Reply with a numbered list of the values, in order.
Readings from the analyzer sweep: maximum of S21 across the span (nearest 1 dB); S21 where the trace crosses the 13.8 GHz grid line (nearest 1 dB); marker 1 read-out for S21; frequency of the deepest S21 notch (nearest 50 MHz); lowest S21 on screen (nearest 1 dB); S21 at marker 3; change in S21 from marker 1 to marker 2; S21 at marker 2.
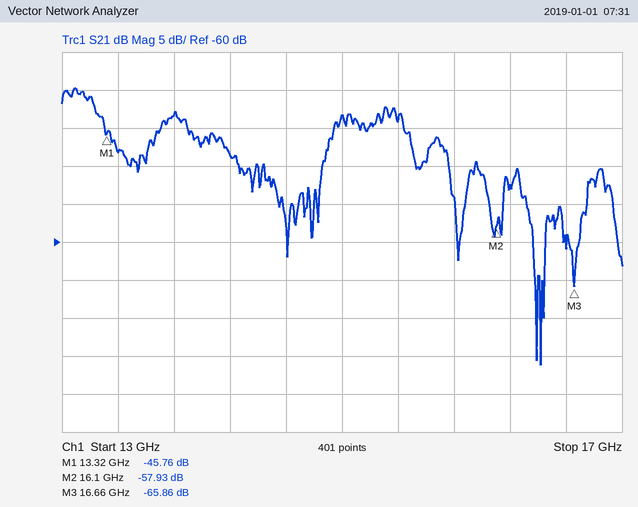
1. -40 dB
2. -43 dB
3. -45.76 dB
4. 16.40 GHz
5. -76 dB
6. -65.86 dB
7. -12.17 dB
8. -57.93 dB
